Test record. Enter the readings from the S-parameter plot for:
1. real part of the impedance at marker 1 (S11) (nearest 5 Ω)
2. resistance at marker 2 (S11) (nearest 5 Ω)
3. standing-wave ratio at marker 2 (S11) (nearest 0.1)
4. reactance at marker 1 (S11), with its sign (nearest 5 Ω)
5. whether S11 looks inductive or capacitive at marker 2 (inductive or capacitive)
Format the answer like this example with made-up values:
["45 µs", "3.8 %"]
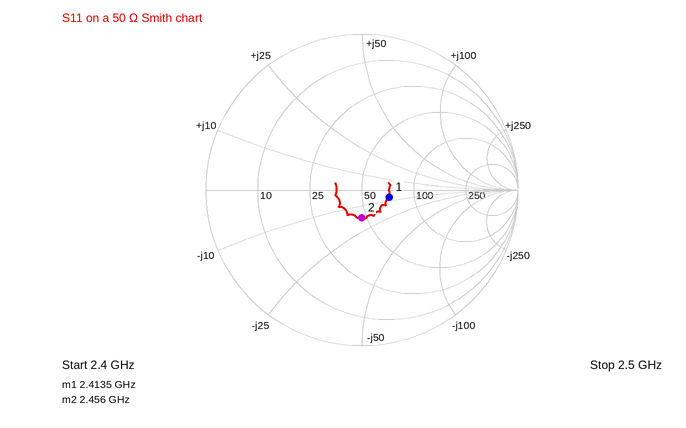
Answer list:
["70 Ω", "45 Ω", "1.4", "-5 Ω", "capacitive"]
